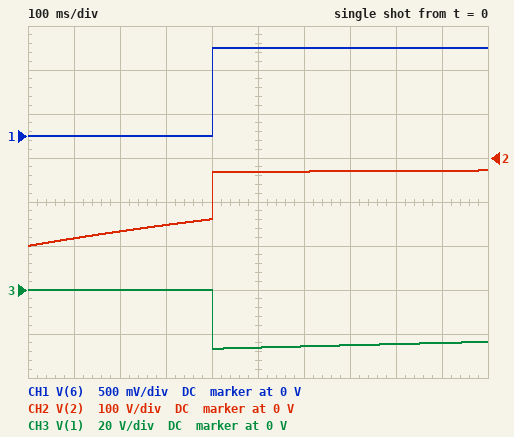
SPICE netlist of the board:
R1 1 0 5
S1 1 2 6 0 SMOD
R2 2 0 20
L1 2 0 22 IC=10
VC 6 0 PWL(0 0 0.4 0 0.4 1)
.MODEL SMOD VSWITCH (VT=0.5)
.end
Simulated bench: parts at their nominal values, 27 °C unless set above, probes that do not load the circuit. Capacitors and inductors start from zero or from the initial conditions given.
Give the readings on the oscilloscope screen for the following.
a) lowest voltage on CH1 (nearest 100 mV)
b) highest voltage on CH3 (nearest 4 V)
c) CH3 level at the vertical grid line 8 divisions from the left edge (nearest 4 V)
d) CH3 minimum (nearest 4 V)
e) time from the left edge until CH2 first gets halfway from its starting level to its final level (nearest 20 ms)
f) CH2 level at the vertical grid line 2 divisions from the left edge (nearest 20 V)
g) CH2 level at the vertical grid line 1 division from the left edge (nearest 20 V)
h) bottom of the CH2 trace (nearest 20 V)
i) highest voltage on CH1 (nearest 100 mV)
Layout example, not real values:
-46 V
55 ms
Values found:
0 V
0 V
-24 V
-28 V
400 ms
-160 V
-180 V
-200 V
1.0 V
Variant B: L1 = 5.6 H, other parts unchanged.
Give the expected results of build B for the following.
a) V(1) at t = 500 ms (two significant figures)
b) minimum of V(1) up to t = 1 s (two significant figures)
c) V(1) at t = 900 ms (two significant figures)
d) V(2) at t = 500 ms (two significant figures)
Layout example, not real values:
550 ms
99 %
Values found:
-8.5 V
-9.2 V
-6.1 V
-10 V
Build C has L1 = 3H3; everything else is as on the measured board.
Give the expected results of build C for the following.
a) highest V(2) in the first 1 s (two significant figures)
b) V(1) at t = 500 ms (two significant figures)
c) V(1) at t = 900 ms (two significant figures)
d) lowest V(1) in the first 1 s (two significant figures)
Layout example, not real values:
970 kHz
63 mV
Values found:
-1.8 V
-3.0 V
-1.7 V
-3.4 V
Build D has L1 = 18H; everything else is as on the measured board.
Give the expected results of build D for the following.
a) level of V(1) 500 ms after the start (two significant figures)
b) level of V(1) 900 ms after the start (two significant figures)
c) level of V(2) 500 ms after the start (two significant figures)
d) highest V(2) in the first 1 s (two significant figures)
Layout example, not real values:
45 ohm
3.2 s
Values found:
-24 V
-22 V
-29 V
-25 V
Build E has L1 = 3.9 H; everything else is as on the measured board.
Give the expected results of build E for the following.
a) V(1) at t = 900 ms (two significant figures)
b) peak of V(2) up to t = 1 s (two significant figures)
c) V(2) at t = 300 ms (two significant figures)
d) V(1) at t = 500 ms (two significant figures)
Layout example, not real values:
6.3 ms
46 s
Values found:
-2.7 V
-2.9 V
-43 V
-4.4 V
